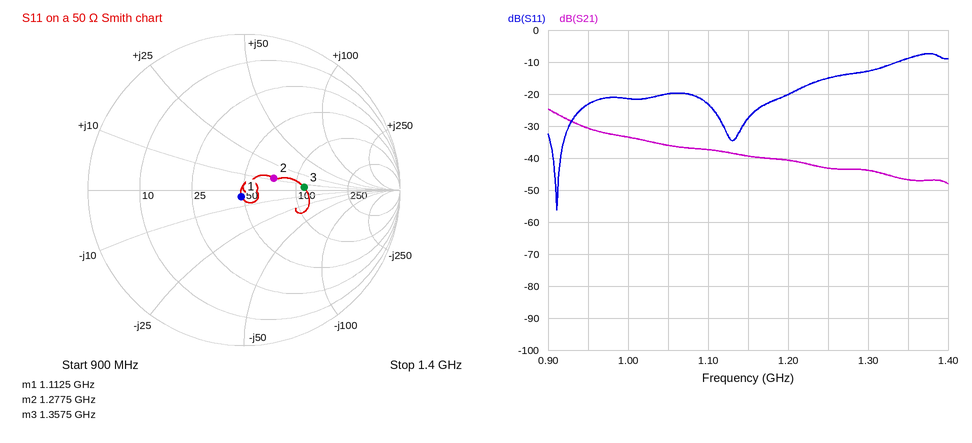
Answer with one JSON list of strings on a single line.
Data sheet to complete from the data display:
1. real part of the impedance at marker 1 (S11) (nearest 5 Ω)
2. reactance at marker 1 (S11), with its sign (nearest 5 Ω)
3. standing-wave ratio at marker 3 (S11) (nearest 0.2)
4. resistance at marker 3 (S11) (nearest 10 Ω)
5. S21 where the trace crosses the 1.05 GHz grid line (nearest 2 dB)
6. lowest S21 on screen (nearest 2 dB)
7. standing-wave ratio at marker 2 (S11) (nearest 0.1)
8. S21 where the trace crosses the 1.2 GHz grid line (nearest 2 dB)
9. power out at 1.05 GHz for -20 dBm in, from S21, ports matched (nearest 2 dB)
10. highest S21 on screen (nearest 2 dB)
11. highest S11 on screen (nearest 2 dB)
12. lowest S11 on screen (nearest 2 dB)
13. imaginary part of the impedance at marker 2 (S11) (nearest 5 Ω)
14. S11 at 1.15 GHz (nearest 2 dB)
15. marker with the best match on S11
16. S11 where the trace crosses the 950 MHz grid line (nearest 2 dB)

["50 Ω", "-5 Ω", "2.2", "110 Ω", "-36 dB", "-48 dB", "1.5", "-40 dB", "-56 dBm", "-24 dB", "-8 dB", "-56 dB", "+10 Ω", "-28 dB", "marker 1", "-24 dB"]
